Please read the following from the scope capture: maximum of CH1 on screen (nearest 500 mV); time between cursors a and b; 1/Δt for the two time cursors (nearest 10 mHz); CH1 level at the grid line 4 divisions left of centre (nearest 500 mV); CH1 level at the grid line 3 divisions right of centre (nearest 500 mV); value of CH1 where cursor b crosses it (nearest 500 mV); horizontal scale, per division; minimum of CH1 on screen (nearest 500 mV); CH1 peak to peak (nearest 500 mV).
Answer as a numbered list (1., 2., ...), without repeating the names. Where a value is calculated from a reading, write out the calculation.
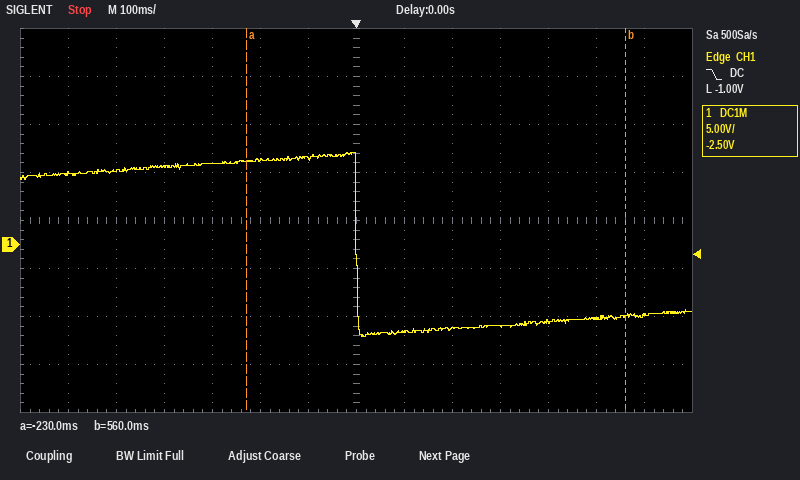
1. 9.5 V
2. 560 ms − (-230 ms) = 790 ms
3. 1 / 790 ms ≈ 1.27 Hz
4. 8.0 V
5. -8.5 V
6. -7.5 V
7. 100 ms
8. -9.5 V
9. 9.5 V − (-9.5 V) = 19.0 V
